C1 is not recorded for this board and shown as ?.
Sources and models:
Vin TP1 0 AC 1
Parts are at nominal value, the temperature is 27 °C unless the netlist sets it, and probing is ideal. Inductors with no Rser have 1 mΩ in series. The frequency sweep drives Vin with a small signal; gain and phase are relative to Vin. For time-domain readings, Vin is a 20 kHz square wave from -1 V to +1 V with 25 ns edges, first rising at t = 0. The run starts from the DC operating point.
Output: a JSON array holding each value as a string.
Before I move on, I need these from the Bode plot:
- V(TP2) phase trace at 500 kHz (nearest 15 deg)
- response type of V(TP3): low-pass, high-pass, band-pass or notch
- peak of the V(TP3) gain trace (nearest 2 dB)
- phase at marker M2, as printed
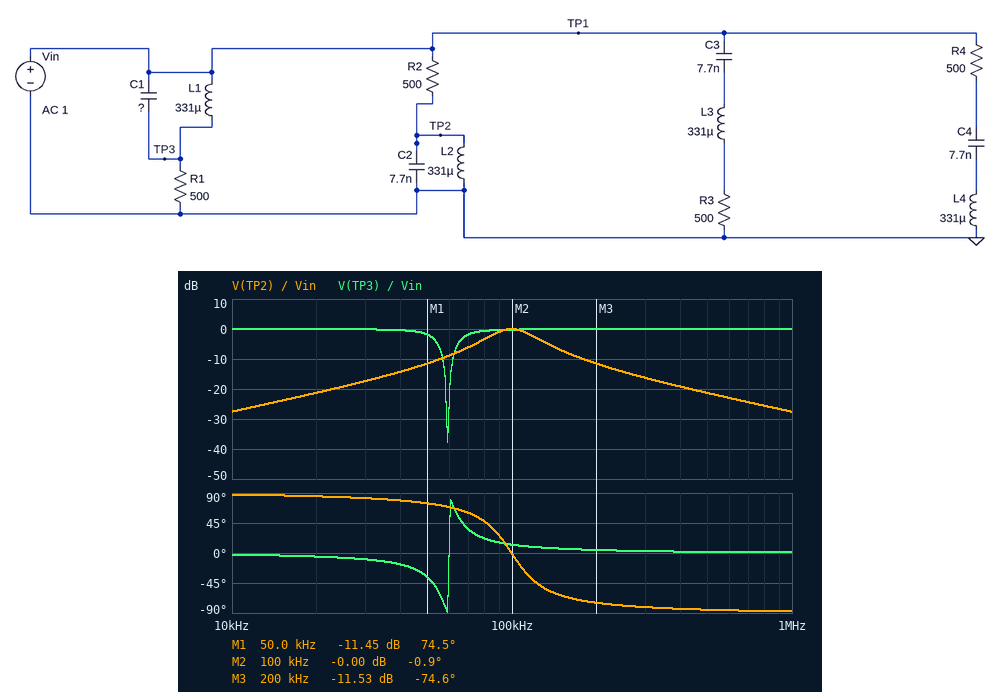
["-90 deg", "notch", "0 dB", "-0.9 deg"]
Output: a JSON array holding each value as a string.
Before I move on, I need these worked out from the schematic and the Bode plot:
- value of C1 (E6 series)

["22 nF"]
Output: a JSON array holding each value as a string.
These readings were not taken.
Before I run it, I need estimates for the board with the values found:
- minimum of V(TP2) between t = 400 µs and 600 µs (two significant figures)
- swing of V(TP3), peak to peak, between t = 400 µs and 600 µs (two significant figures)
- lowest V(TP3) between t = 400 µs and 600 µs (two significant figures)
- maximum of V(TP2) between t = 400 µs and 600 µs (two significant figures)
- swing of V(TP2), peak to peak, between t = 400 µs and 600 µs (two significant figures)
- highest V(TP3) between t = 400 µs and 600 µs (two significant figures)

["-640 mV", "2.8 V", "-1.4 V", "640 mV", "1.3 V", "1.4 V"]
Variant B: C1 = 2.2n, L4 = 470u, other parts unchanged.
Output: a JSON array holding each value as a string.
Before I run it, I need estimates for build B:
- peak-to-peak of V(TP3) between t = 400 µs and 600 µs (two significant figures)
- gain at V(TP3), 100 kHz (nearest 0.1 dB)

["2.5 V", "-1.3 dB"]
